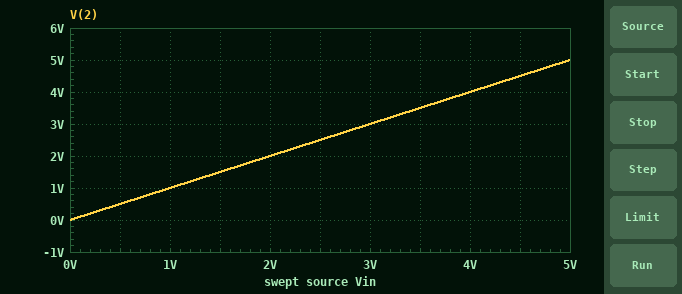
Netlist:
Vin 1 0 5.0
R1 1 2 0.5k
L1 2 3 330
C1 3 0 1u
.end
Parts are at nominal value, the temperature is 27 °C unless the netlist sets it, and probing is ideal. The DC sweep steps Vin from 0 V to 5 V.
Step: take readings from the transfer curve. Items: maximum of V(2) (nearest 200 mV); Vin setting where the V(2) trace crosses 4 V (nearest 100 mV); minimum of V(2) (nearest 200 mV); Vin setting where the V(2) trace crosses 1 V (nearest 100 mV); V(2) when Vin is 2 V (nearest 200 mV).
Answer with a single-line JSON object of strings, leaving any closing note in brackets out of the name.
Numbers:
{"maximum of V(2)": "5.0 V", "Vin setting where the V(2) trace crosses 4 V": "4.0 V", "minimum of V(2)": "0 V", "Vin setting where the V(2) trace crosses 1 V": "1.0 V", "V(2) when Vin is 2 V": "2.0 V"}
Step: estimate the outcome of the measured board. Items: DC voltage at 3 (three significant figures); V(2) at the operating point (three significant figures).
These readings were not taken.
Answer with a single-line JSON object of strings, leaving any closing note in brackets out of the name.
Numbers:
{"DC voltage at 3": "5.00 V", "V(2) at the operating point": "5.00 V"}
